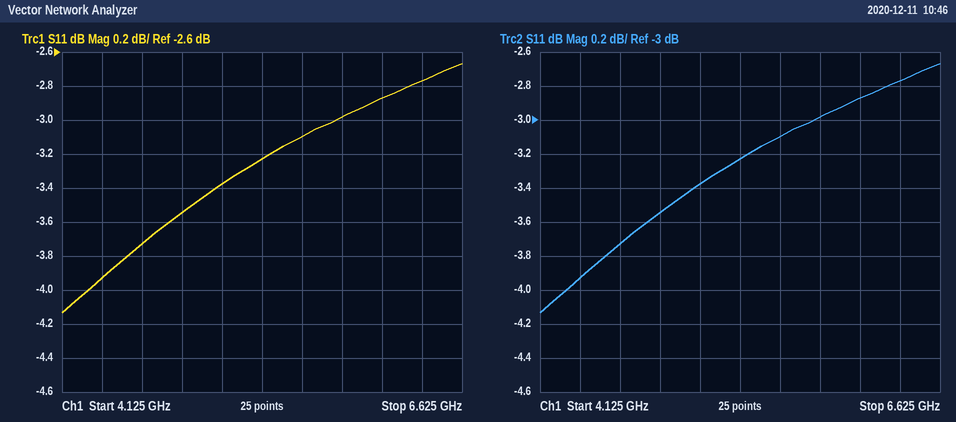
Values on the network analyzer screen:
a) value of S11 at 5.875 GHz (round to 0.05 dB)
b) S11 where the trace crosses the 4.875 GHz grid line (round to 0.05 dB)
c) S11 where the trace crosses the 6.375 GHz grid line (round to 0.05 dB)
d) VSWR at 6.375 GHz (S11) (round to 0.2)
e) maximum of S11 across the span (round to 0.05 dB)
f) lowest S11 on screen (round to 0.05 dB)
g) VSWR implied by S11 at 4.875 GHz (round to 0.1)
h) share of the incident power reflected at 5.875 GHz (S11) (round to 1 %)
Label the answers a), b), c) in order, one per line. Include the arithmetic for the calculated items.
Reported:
a) -3.00 dB
b) -3.55 dB
c) -2.75 dB
d) |Γ| = 10^(-2.75/20) = 0.7286; VSWR = (1 + 0.7286)/(1 − 0.7286) ≈ 6.4
e) -2.65 dB
f) -4.15 dB
g) |Γ| = 10^(-3.55/20) = 0.6645; VSWR = (1 + 0.6645)/(1 − 0.6645) ≈ 5.0
h) 10^(-3/10) ≈ 50 %
